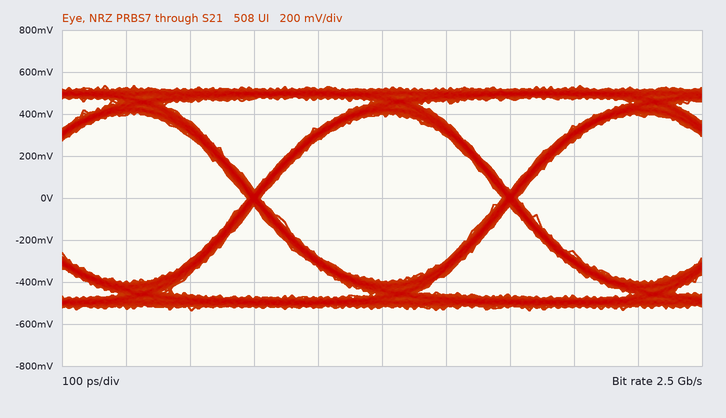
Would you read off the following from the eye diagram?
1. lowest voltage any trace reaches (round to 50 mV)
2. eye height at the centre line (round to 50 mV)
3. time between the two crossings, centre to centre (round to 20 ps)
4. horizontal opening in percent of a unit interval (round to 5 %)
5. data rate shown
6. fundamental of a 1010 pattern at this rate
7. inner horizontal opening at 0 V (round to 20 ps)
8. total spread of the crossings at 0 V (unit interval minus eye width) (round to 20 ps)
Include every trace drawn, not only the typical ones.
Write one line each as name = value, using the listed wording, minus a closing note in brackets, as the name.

lowest voltage any trace reaches = -550 mV
eye height at the centre line = 800 mV
time between the two crossings, centre to centre = 400 ps
horizontal opening in percent of a unit interval = 95 %
data rate shown = 2.5 Gb/s
fundamental of a 1010 pattern at this rate = 1.25 GHz
inner horizontal opening at 0 V = 380 ps
total spread of the crossings at 0 V (unit interval minus eye width) = 20 ps
